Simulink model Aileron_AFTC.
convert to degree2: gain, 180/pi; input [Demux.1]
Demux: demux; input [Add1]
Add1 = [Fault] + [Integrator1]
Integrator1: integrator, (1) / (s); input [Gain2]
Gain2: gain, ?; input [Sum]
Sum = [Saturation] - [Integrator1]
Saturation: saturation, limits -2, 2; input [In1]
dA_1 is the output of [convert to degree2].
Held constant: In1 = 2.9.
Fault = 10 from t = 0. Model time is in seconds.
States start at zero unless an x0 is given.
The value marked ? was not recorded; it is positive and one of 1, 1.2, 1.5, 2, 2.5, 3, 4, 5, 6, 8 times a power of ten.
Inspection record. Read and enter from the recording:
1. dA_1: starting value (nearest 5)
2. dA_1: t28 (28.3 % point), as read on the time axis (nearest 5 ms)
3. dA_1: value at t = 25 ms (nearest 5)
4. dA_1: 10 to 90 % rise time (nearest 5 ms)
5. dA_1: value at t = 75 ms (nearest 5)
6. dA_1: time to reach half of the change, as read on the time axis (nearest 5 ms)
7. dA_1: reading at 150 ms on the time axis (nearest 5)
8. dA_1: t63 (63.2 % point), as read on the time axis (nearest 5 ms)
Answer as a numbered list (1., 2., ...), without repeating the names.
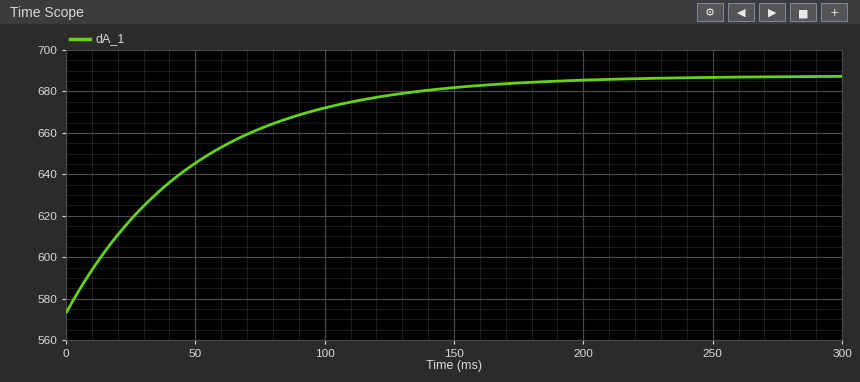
1. 575
2. 15 ms
3. 620
4. 110 ms
5. 660
6. 35 ms
7. 680
8. 50 ms
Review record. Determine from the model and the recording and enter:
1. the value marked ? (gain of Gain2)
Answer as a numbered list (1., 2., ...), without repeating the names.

1. 20
